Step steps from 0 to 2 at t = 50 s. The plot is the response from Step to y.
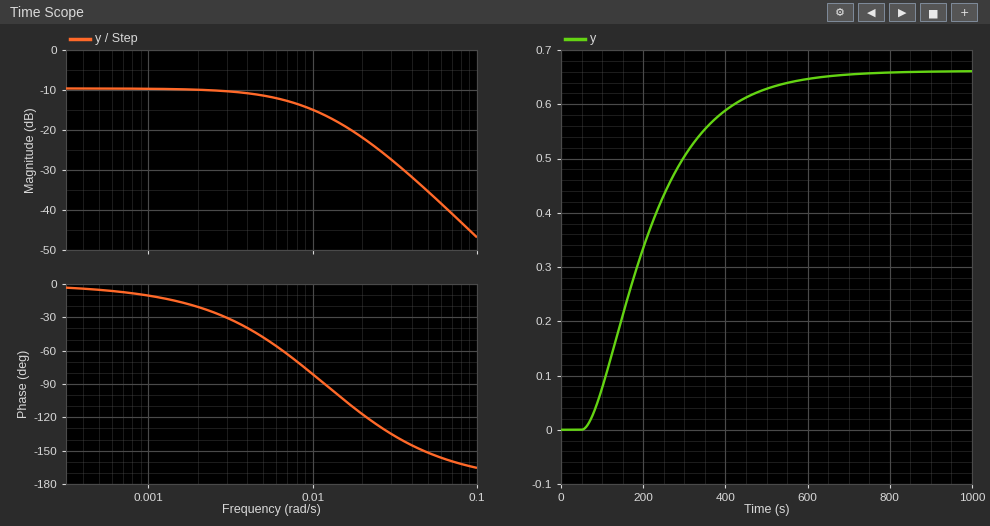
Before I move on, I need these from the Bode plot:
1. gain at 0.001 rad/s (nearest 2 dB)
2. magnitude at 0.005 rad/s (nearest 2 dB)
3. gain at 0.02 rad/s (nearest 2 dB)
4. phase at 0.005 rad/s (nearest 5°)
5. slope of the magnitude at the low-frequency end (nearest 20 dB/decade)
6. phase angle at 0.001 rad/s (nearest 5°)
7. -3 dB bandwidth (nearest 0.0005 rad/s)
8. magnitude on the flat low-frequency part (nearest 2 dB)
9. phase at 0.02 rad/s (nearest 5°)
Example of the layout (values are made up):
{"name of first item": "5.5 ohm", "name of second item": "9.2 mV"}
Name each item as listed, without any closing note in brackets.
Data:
{"gain at 0.001 rad/s": "-10 dB", "magnitude at 0.005 rad/s": "-12 dB", "gain at 0.02 rad/s": "-22 dB", "phase at 0.005 rad/s": "-50°", "slope of the magnitude at the low-frequency end": "0 dB/decade", "phase angle at 0.001 rad/s": "-10°", "-3 dB bandwidth": "0.0070 rad/s", "magnitude on the flat low-frequency part": "-10 dB", "phase at 0.02 rad/s": "-115°"}
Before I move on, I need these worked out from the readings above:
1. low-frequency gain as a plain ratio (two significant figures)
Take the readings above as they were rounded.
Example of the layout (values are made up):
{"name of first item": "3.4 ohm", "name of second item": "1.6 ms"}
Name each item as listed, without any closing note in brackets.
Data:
{"low-frequency gain as a plain ratio": "0.32"}
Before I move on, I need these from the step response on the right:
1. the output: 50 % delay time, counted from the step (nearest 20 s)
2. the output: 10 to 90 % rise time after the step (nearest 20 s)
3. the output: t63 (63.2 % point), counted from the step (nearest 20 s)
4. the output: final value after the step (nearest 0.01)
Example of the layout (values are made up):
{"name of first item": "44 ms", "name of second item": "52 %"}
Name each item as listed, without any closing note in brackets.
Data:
{"the output: 50 % delay time, counted from the step": "140 s", "the output: 10 to 90 % rise time after the step": "320 s", "the output: t63 (63.2 % point), counted from the step": "200 s", "the output: final value after the step": "0.66"}
